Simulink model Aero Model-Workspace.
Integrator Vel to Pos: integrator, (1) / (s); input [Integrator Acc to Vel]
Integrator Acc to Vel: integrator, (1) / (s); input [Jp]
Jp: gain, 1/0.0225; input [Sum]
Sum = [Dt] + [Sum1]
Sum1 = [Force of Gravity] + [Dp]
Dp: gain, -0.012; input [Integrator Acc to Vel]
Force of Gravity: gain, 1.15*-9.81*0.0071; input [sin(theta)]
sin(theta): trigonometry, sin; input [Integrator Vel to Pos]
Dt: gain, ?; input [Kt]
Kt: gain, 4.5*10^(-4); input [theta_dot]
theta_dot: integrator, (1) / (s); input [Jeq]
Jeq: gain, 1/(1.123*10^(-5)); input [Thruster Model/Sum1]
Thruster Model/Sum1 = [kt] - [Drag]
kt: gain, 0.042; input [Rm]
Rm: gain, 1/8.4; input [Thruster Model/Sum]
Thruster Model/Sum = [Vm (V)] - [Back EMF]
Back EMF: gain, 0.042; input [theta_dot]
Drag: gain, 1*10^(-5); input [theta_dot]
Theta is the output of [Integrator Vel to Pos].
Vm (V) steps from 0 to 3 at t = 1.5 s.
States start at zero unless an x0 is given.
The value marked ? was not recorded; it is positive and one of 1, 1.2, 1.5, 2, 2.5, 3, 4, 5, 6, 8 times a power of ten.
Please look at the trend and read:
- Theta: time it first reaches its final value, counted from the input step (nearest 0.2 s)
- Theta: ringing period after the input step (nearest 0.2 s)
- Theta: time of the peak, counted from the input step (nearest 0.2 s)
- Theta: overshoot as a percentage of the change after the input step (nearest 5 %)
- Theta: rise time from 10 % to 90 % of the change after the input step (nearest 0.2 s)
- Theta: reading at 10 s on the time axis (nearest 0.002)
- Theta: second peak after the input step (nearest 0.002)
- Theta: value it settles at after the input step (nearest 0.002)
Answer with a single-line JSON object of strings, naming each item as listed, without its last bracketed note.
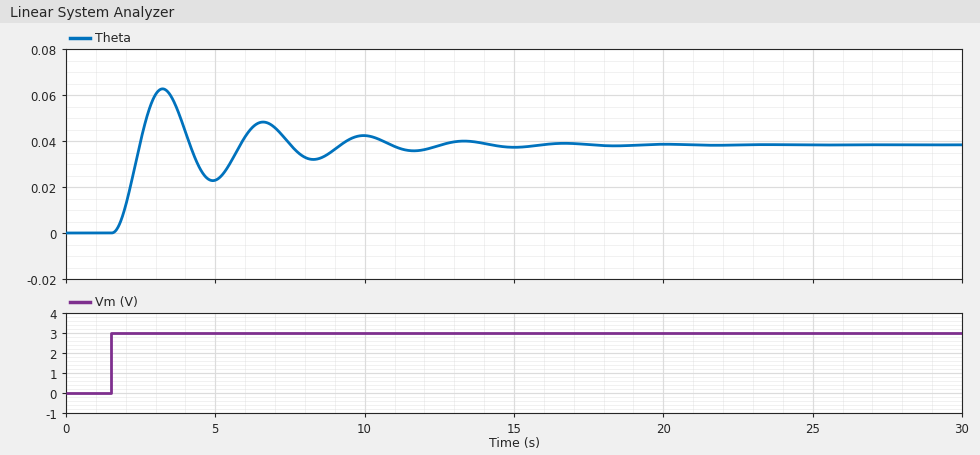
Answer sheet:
{"Theta: time it first reaches its final value, counted from the input step": "1.0 s", "Theta: ringing period after the input step": "3.4 s", "Theta: time of the peak, counted from the input step": "1.8 s", "Theta: overshoot as a percentage of the change after the input step": "65 %", "Theta: rise time from 10 % to 90 % of the change after the input step": "0.6 s", "Theta: reading at 10 s on the time axis": "0.042", "Theta: second peak after the input step": "0.048", "Theta: value it settles at after the input step": "0.038"}
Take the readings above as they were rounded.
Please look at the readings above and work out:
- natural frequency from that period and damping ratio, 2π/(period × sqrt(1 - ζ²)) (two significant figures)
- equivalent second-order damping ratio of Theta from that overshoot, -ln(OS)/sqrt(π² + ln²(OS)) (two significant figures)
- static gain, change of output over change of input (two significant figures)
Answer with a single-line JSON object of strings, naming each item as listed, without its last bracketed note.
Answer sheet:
{"natural frequency from that period and damping ratio, 2π/(period × sqrt(1 - ζ²))": "1.9 rad/s", "equivalent second-order damping ratio of Theta from that overshoot, -ln(OS)/sqrt(π² + ln²(OS))": "0.14", "static gain, change of output over change of input": "0.013"}
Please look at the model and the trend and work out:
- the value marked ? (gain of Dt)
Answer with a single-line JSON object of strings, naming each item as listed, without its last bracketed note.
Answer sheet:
{"the value marked ?": "0.1"}
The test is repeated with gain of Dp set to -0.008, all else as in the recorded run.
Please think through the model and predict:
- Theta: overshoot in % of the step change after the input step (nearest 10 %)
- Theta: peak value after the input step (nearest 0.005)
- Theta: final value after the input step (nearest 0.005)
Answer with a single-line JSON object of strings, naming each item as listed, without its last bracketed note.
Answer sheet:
{"Theta: overshoot in % of the step change after the input step": "70 %", "Theta: peak value after the input step": "0.065", "Theta: final value after the input step": "0.040"}
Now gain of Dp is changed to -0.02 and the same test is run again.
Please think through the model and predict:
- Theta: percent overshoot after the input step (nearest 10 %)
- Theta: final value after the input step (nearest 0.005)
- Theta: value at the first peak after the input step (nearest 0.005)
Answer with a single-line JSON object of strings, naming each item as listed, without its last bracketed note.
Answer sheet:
{"Theta: percent overshoot after the input step": "50 %", "Theta: final value after the input step": "0.040", "Theta: value at the first peak after the input step": "0.055"}
